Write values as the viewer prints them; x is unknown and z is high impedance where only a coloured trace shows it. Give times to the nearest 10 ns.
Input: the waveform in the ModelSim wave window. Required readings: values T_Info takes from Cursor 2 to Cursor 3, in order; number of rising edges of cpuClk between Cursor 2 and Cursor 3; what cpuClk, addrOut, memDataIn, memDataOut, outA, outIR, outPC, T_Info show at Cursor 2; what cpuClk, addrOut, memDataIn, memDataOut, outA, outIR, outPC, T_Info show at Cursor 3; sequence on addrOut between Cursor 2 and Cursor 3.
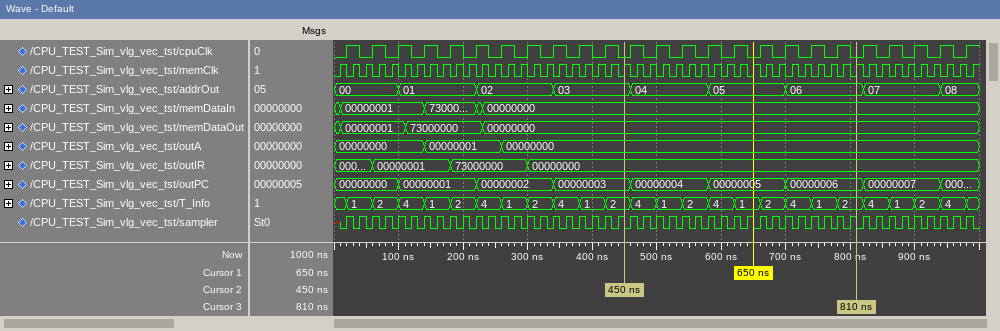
2, 4, 1, 2, 4, 1, 2, 4, 1, 2
9
cpuClk=0, addrOut=03, memDataIn=00000000, memDataOut=00000000, outA=00000000, outIR=00000000, outPC=00000003, T_Info=2
cpuClk=0, addrOut=06, memDataIn=00000000, memDataOut=00000000, outA=00000000, outIR=00000000, outPC=00000006, T_Info=2
03, 04, 05, 06
